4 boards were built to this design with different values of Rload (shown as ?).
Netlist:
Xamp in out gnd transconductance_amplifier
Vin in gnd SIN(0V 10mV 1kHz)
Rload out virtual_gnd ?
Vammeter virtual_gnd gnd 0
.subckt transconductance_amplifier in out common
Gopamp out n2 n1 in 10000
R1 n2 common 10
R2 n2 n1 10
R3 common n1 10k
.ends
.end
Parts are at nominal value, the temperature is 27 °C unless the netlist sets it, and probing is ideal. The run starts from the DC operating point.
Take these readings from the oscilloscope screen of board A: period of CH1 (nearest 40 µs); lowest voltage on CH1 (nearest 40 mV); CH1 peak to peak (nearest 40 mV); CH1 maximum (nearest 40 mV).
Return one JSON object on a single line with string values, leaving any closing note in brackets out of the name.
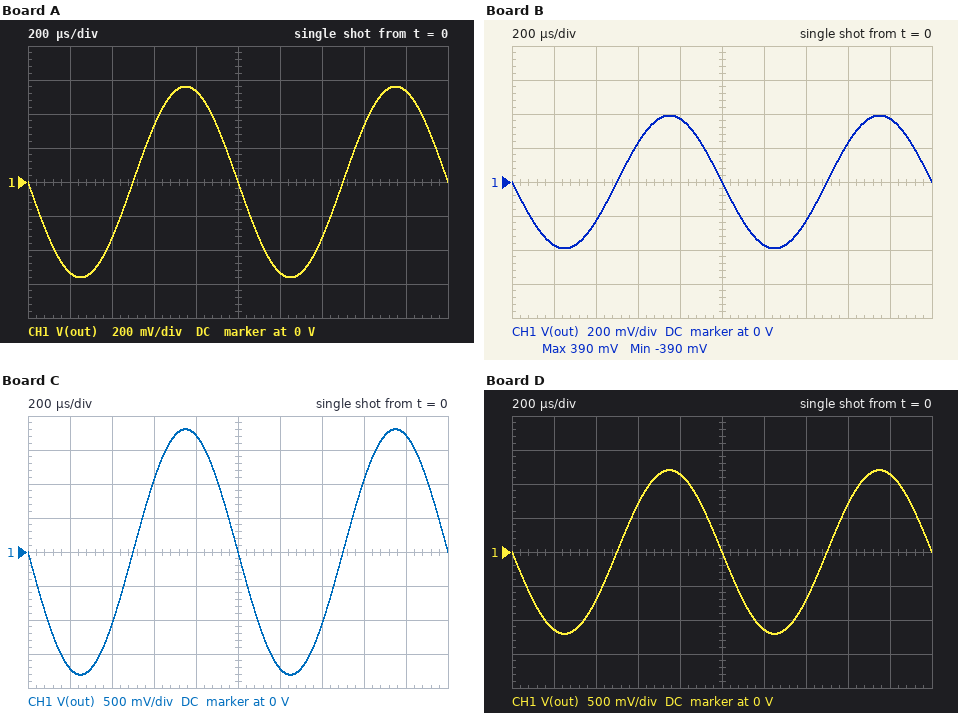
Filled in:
{"period of CH1": "1.00 ms", "lowest voltage on CH1": "-560 mV", "CH1 peak to peak": "1.12 V", "CH1 maximum": "560 mV"}
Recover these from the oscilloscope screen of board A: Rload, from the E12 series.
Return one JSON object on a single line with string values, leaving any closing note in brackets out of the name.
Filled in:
{"Rload, from the E12 series": "560 Ω"}
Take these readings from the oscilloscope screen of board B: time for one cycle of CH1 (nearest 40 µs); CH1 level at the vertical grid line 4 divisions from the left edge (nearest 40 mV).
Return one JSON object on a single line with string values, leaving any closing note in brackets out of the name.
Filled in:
{"time for one cycle of CH1": "1.00 ms", "CH1 level at the vertical grid line 4 divisions from the left edge": "360 mV"}
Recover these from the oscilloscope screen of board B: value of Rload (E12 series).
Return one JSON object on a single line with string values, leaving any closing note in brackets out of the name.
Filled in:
{"value of Rload": "390 Ω"}
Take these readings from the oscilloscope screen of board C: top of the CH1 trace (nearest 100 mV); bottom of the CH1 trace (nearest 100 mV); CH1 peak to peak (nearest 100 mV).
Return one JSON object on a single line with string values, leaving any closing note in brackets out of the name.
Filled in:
{"top of the CH1 trace": "1.8 V", "bottom of the CH1 trace": "-1.8 V", "CH1 peak to peak": "3.6 V"}
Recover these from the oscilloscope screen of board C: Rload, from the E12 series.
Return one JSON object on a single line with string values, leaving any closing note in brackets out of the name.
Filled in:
{"Rload, from the E12 series": "1.8 kΩ"}
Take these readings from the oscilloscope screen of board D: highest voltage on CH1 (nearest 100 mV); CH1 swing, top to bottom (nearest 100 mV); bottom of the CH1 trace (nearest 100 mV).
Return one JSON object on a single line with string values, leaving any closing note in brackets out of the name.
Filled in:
{"highest voltage on CH1": "1.2 V", "CH1 swing, top to bottom": "2.4 V", "bottom of the CH1 trace": "-1.2 V"}
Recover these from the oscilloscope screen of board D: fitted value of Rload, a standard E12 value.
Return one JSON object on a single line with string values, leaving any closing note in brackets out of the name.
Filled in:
{"fitted value of Rload, a standard E12 value": "1.2 kΩ"}
